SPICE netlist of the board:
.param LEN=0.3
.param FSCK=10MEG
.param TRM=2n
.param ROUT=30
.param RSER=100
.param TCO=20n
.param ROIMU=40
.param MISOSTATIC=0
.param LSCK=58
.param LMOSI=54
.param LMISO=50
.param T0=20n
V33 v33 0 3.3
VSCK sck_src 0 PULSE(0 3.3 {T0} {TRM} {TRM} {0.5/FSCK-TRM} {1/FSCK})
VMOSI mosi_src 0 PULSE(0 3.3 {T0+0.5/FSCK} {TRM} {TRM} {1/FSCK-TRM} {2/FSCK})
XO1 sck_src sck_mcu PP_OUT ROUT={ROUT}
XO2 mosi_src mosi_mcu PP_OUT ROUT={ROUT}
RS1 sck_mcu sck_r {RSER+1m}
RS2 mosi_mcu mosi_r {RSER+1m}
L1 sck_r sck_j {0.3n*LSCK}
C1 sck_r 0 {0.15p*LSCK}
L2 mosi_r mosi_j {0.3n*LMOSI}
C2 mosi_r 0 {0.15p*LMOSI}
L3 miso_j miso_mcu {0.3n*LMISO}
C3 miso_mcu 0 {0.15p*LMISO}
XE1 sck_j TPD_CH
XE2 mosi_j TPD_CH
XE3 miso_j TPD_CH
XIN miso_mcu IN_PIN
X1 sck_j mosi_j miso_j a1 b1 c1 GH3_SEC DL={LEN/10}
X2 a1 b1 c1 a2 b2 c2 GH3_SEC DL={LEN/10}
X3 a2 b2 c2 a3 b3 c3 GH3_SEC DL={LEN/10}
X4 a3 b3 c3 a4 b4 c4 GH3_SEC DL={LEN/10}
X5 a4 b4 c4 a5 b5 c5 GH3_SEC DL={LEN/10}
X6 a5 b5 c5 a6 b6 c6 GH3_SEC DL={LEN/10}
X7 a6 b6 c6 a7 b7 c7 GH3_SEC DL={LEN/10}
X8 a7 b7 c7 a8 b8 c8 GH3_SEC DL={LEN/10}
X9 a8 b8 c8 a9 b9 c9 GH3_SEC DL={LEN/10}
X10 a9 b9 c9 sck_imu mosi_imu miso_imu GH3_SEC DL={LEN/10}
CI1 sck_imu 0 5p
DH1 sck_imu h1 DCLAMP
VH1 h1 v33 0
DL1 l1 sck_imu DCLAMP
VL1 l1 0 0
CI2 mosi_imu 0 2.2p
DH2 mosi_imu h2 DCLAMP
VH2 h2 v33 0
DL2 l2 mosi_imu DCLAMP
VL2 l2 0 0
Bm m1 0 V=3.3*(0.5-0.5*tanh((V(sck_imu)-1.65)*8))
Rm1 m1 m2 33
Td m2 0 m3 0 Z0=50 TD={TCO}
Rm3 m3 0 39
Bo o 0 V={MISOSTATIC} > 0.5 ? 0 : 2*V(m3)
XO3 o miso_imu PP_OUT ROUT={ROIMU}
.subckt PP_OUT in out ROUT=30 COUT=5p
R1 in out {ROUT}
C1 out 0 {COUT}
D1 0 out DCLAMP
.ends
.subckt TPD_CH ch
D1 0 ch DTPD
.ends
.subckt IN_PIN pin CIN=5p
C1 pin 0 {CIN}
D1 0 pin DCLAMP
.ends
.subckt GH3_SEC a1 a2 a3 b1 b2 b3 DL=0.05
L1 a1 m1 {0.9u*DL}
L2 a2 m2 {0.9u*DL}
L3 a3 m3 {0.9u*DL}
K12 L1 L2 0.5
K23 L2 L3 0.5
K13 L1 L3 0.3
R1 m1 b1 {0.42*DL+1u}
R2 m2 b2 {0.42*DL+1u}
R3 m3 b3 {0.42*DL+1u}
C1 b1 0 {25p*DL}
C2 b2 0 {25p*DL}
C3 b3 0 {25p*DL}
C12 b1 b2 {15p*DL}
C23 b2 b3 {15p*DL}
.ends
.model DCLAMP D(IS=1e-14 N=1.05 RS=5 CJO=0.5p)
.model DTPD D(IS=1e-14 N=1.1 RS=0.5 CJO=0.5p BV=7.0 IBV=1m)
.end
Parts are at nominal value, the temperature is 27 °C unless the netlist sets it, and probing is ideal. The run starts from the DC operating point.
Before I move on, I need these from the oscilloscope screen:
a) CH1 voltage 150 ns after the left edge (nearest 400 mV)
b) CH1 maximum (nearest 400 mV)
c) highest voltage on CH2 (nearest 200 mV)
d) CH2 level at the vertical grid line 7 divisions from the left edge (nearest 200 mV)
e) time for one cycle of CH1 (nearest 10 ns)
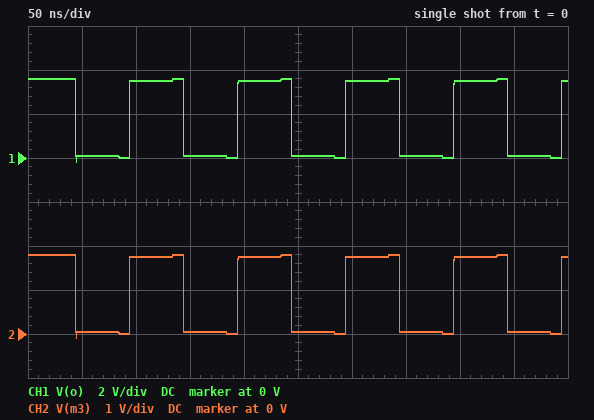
0 V
3.6 V
1.8 V
0 V
100 ns
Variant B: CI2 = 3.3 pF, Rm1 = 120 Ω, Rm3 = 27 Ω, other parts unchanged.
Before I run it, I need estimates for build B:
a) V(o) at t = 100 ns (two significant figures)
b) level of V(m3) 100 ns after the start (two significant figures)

1.4 V
690 mV
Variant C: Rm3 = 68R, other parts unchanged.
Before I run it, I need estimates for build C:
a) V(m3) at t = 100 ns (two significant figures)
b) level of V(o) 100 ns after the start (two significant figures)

2.3 V
4.6 V
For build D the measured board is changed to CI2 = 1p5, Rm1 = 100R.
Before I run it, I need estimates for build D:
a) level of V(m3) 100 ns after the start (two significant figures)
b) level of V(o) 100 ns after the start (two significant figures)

970 mV
1.9 V
